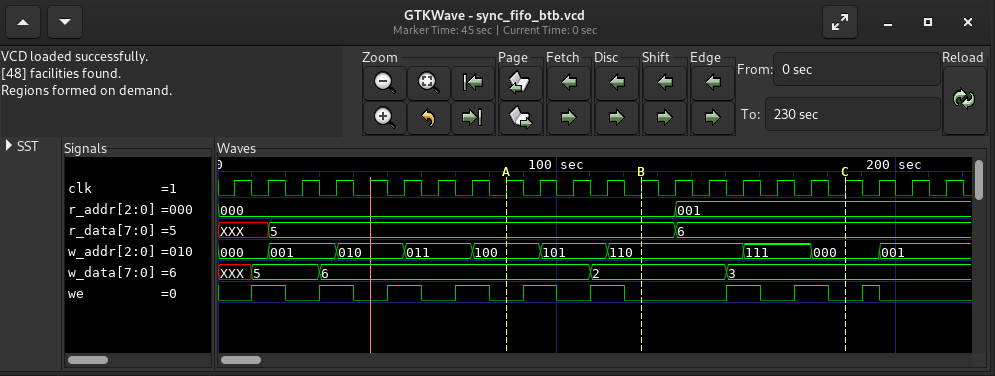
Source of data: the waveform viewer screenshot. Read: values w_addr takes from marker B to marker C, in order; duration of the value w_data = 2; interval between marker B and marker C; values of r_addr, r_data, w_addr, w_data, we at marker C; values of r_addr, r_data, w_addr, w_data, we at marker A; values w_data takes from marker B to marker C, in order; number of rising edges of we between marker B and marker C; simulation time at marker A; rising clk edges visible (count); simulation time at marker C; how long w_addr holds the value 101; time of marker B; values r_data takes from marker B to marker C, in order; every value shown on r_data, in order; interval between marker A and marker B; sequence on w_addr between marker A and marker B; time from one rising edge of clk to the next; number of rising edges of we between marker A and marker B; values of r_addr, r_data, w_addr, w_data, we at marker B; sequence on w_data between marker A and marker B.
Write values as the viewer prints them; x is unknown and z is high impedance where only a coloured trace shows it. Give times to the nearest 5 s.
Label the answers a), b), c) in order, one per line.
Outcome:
a) 110, 111, 000
b) 40 s
c) 60 s
d) r_addr=001, r_data=6, w_addr=000, w_data=3, we=0
e) r_addr=000, r_data=5, w_addr=100, w_data=6, we=0
f) 2, 3
g) 2
h) 85 s
i) 22
j) 185 s
k) 20 s
l) 125 s
m) 5, 6
n) XXX, 5, 6
o) 40 s
p) 100, 101, 110
q) 10 s
r) 2
s) r_addr=000, r_data=5, w_addr=110, w_data=2, we=0
t) 6, 2
